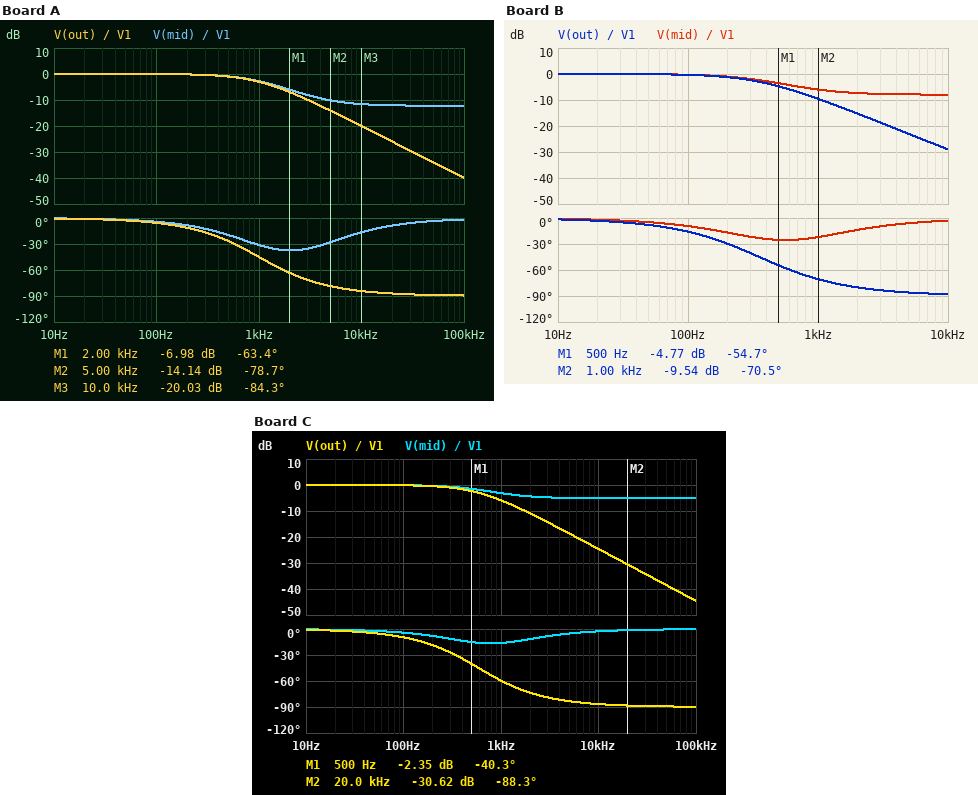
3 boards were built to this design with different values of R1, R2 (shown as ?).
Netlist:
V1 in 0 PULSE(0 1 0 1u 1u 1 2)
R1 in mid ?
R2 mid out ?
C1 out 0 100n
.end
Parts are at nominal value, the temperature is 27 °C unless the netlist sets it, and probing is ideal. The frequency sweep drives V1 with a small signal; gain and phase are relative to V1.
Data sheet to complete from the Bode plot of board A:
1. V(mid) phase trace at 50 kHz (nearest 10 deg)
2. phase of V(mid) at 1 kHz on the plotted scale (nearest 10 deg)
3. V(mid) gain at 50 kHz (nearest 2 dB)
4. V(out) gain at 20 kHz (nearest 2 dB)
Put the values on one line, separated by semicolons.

0 deg; -30 deg; -12 dB; -26 dB
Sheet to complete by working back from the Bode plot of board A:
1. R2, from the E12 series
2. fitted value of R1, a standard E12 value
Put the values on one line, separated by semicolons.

390 Ω; 1.2 kΩ
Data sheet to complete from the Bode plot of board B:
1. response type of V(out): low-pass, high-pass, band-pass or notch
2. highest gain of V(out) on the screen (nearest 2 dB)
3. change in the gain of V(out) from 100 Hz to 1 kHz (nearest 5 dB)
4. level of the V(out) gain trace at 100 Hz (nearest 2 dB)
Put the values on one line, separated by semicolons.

low-pass; 0 dB; -10 dB; 0 dB
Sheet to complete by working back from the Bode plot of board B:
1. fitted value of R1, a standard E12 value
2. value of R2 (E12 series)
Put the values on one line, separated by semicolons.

2.7 kΩ; 1.8 kΩ
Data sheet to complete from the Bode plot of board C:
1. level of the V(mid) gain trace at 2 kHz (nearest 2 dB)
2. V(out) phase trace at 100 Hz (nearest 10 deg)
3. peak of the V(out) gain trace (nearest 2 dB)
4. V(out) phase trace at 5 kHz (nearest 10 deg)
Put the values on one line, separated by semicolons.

-4 dB; -10 deg; 0 dB; -80 deg
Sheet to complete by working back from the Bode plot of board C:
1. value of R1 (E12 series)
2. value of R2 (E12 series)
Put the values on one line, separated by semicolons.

1.2 kΩ; 1.5 kΩ
